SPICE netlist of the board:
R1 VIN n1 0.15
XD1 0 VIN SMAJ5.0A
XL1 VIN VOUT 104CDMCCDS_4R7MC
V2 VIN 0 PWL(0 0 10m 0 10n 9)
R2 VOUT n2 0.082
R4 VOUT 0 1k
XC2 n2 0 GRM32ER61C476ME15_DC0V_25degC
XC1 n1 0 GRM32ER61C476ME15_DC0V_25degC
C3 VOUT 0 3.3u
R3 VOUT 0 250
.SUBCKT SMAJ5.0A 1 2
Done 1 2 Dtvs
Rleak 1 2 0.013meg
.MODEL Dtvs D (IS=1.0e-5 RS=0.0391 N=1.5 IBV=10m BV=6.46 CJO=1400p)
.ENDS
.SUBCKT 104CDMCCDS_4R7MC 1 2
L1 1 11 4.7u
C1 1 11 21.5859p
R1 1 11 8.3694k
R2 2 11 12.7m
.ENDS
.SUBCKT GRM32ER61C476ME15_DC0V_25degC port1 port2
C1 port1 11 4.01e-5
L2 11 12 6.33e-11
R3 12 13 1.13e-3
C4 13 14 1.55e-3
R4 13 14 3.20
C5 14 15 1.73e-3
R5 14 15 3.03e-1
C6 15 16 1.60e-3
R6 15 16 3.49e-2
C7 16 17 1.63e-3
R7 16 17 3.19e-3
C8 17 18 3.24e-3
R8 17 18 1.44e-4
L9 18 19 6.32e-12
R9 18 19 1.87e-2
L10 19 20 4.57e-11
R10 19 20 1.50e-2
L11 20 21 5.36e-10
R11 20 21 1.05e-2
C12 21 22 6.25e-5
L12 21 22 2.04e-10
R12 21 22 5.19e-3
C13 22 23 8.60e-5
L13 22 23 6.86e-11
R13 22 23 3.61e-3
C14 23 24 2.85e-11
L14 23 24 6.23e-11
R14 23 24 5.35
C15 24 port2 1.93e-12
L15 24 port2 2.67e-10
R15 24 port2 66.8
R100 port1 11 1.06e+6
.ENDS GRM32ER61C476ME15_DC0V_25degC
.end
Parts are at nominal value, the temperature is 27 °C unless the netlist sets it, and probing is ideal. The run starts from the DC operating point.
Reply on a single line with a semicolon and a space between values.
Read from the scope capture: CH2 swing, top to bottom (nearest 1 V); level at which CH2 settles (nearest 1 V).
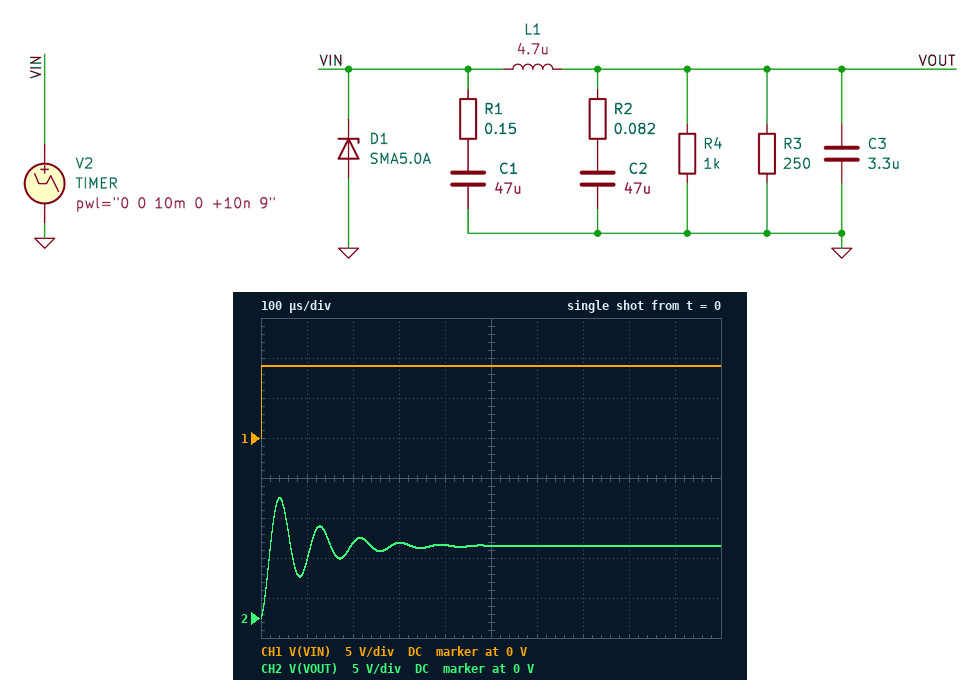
15 V; 9 V
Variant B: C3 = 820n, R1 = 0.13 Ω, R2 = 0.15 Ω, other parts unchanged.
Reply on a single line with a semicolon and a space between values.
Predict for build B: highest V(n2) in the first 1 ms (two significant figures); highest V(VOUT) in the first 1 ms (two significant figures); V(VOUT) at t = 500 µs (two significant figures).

13 V; 14 V; 9.0 V
